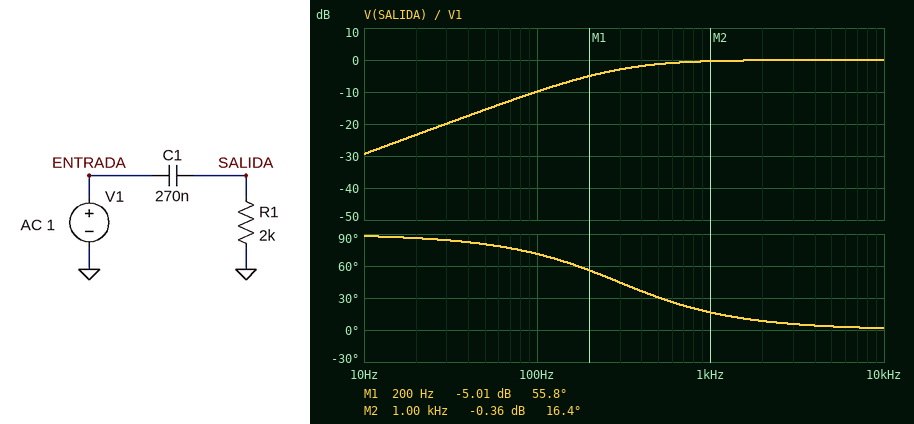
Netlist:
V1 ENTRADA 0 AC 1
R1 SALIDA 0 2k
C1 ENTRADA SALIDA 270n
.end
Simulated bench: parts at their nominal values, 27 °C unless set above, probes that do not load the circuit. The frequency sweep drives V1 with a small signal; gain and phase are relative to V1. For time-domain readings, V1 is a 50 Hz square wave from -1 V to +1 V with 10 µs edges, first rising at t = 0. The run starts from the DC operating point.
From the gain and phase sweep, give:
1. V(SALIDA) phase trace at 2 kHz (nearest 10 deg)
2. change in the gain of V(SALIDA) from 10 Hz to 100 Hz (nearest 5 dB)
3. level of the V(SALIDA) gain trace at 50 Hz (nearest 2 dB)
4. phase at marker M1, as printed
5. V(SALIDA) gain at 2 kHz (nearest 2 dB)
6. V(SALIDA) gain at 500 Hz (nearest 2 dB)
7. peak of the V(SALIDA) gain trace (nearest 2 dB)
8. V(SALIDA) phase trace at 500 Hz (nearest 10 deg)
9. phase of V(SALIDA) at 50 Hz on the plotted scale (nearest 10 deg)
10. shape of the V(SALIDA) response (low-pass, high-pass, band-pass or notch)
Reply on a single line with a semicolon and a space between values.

10 deg; 20 dB; -16 dB; 55.8 deg; 0 dB; -2 dB; 0 dB; 30 deg; 80 deg; high-pass
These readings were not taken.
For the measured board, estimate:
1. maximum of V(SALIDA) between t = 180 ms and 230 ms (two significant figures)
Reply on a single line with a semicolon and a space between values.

2.0 V
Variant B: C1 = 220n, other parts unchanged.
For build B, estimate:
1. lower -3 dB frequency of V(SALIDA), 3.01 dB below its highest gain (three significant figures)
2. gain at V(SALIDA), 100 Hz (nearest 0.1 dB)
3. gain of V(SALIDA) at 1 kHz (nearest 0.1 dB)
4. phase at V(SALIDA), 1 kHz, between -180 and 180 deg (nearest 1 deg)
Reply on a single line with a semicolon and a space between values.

362 Hz; -11.5 dB; -0.5 dB; 20 deg
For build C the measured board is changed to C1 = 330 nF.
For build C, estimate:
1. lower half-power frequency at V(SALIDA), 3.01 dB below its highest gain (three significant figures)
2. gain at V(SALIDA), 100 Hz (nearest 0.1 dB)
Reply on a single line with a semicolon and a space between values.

241 Hz; -8.3 dB
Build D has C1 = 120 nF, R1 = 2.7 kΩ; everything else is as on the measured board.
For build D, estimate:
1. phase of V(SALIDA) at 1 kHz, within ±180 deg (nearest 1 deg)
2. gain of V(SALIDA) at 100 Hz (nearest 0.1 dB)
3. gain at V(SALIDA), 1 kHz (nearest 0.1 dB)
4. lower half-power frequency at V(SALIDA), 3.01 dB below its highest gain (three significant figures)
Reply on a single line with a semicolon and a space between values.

26 deg; -14.0 dB; -0.9 dB; 491 Hz
